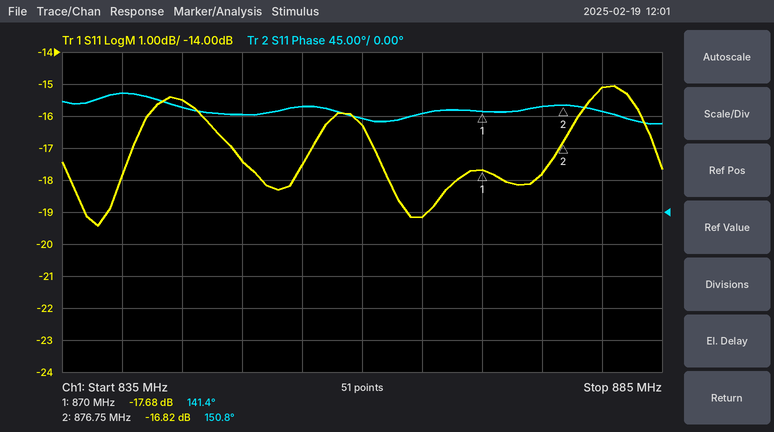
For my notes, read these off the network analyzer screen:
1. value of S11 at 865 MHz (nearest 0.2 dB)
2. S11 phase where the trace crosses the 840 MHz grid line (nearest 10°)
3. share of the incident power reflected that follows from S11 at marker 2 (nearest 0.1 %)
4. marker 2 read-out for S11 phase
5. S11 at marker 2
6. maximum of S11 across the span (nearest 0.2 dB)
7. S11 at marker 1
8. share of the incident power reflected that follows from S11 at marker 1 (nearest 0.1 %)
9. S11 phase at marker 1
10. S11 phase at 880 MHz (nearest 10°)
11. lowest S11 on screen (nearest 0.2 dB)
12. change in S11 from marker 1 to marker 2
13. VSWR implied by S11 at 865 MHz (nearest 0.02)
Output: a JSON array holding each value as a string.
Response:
["-19.2 dB", "170°", "2.1 %", "150.8°", "-16.82 dB", "-15.0 dB", "-17.68 dB", "1.7 %", "141.4°", "140°", "-19.4 dB", "0.86 dB", "1.24"]
